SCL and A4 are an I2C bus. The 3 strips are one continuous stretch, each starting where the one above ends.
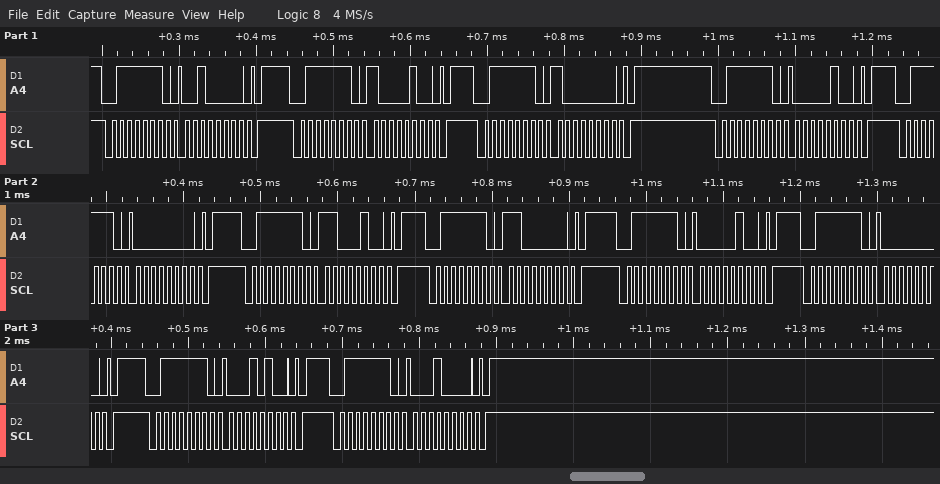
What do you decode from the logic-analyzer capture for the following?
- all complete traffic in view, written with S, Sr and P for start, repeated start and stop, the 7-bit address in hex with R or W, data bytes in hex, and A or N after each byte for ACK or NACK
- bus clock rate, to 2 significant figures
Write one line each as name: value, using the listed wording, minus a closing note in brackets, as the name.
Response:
all complete traffic in view, written with S, Sr and P for start, repeated start and stop, the 7-bit address in hex with R or W, data bytes in hex, and A or N after each byte for ACK or NACK: S 3FW A 20 A P S 3FW A 84 A P S 3FW A 80 A P S 3FW A 04 A P S 3FW A 00 A P S 3FW A C4 A P S 3FW A C0 A P S 3FW A 04 A P S 3FW A 00 A P S 3FW A 14 A P S 3FW A 10 A P
bus clock rate, to 2 significant figures: 100 kHz
